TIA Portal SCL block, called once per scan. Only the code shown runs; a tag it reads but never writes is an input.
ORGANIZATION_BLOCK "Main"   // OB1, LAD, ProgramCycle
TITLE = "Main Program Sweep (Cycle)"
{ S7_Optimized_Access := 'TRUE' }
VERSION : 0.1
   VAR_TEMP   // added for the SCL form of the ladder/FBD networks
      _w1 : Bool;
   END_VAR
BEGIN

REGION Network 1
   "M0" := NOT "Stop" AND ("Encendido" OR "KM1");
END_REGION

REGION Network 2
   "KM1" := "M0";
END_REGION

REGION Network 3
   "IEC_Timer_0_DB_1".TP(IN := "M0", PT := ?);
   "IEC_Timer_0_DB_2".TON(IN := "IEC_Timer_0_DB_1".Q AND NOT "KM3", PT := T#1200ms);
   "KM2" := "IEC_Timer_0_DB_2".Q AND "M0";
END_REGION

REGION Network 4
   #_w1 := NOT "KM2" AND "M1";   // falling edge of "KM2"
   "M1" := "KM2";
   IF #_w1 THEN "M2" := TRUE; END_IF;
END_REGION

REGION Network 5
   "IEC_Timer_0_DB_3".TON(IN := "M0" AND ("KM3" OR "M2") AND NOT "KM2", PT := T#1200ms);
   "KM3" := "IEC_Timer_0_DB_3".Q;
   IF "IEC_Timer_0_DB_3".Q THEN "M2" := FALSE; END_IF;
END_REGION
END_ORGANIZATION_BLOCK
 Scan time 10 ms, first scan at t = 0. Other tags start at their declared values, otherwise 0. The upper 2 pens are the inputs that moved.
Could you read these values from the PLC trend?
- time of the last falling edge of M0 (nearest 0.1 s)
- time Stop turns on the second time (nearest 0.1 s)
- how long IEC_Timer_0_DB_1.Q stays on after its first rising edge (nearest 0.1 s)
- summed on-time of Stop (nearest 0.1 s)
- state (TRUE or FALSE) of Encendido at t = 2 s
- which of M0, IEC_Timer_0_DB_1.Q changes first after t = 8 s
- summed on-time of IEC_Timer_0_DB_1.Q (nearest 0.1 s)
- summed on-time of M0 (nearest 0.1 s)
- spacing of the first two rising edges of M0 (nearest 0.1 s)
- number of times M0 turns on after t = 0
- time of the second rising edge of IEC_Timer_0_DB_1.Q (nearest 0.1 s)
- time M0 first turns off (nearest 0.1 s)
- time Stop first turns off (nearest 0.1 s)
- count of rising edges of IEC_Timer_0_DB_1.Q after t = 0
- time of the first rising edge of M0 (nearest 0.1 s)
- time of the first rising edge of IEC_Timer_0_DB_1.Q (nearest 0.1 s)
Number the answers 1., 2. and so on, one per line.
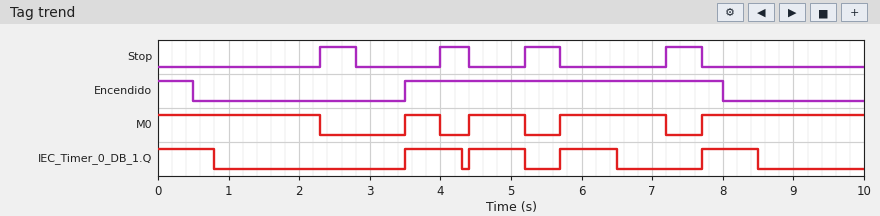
1. 7.2 s
2. 4.0 s
3. 0.8 s
4. 1.9 s
5. FALSE
6. IEC_Timer_0_DB_1.Q
7. 4.0 s
8. 7.4 s
9. 0.9 s
10. 4
11. 4.4 s
12. 2.3 s
13. 2.8 s
14. 4
15. 3.5 s
16. 3.5 s
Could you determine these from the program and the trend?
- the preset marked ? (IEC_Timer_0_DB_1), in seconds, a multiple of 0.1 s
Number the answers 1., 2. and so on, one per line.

1. 0.8 s
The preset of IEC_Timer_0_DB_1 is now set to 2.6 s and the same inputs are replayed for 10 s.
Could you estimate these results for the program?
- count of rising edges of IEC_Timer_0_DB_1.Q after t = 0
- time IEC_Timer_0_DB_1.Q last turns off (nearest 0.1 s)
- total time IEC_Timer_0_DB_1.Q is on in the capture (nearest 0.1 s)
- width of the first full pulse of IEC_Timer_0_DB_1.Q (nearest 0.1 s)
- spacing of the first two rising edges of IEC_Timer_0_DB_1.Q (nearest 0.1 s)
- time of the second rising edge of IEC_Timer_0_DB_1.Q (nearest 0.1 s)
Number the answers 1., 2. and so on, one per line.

1. 2
2. 6.1 s
3. 7.5 s
4. 2.6 s
5. 4.2 s
6. 7.7 s
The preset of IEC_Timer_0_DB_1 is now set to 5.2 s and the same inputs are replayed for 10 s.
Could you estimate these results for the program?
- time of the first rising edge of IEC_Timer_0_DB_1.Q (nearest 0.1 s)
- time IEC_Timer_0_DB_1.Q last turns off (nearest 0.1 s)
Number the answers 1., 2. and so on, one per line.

1. 5.7 s
2. 5.2 s
